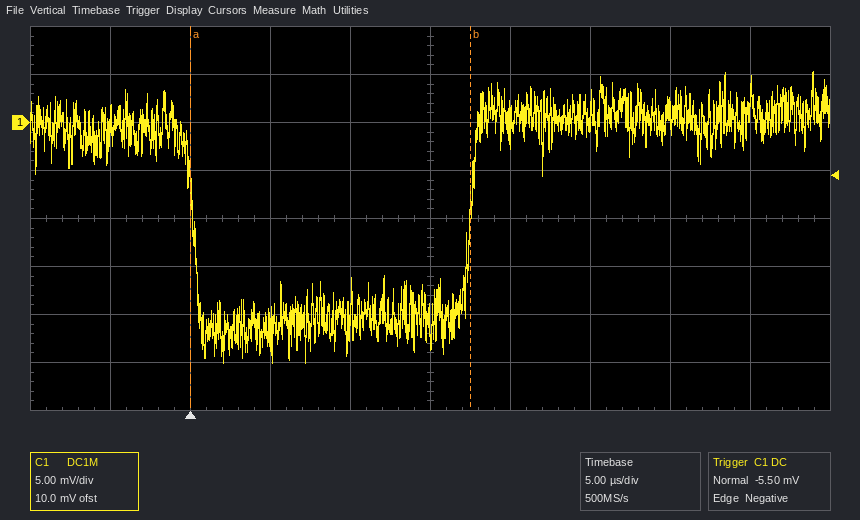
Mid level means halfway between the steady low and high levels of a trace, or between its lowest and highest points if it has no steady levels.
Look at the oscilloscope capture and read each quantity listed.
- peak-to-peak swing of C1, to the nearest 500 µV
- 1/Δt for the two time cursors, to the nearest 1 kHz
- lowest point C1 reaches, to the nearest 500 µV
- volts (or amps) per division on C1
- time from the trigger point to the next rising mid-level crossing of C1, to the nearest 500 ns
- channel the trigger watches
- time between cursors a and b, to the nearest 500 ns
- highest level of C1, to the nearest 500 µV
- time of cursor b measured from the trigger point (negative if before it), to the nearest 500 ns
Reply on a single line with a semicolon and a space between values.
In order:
30.5 mV; 57 kHz; -25.0 mV; 5 mV; 17.5 µs; C1; 17.5 µs; 5.5 mV; +17.5 µs
